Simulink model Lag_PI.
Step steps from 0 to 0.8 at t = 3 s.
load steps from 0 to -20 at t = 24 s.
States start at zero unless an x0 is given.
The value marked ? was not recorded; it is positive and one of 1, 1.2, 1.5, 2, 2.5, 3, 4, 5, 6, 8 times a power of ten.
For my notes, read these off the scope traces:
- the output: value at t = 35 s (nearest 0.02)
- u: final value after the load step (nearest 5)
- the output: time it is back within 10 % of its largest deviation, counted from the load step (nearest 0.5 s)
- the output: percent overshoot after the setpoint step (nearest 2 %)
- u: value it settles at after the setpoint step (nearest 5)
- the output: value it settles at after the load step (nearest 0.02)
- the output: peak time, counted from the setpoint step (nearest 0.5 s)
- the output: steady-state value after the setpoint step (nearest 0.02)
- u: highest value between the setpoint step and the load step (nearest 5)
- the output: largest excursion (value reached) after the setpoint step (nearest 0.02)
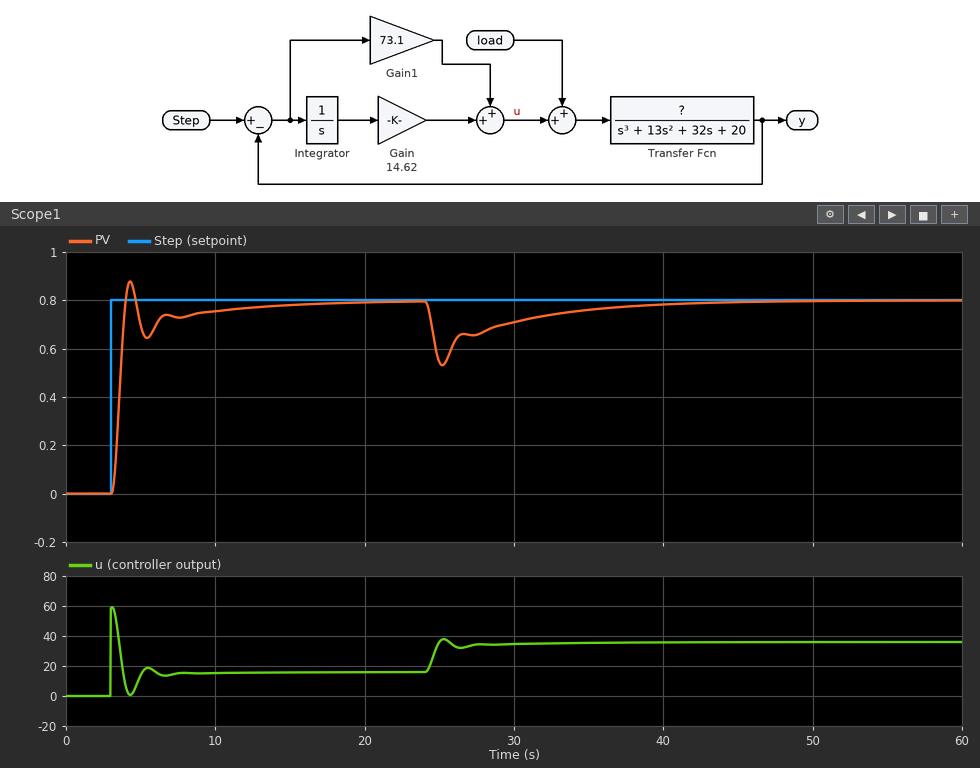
0.76
35
13.5 s
10 %
15
0.80
1.5 s
0.80
60
0.88
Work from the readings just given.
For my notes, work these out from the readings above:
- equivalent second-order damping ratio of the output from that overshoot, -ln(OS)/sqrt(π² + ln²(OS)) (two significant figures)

0.59
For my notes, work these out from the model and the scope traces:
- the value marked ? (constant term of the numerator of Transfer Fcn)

1
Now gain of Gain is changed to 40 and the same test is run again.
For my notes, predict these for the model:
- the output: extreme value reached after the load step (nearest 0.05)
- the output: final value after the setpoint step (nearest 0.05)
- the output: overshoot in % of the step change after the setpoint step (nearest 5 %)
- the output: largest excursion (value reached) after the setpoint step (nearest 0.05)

0.55
0.80
25 %
1.00
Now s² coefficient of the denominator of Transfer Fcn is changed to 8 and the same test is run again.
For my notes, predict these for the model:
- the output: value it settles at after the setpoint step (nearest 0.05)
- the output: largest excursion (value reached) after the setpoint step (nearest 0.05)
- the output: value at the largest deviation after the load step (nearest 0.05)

0.80
0.85
0.55
